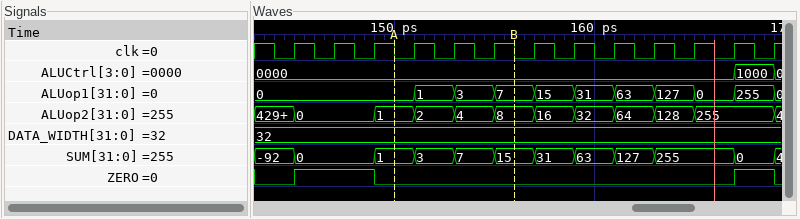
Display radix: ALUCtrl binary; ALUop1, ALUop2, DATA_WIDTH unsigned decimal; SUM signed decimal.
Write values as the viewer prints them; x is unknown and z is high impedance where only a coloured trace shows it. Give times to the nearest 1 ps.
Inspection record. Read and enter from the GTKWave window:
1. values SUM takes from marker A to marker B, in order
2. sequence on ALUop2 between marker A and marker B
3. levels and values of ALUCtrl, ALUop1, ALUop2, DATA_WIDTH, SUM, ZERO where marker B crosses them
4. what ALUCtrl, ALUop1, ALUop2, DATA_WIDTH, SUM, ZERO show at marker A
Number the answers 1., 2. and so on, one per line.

1. 1, 3, 7, 15
2. 1, 2, 4, 8
3. ALUCtrl=0000, ALUop1=7, ALUop2=8, DATA_WIDTH=32, SUM=15, ZERO=0
4. ALUCtrl=0000, ALUop1=0, ALUop2=1, DATA_WIDTH=32, SUM=1, ZERO=0
